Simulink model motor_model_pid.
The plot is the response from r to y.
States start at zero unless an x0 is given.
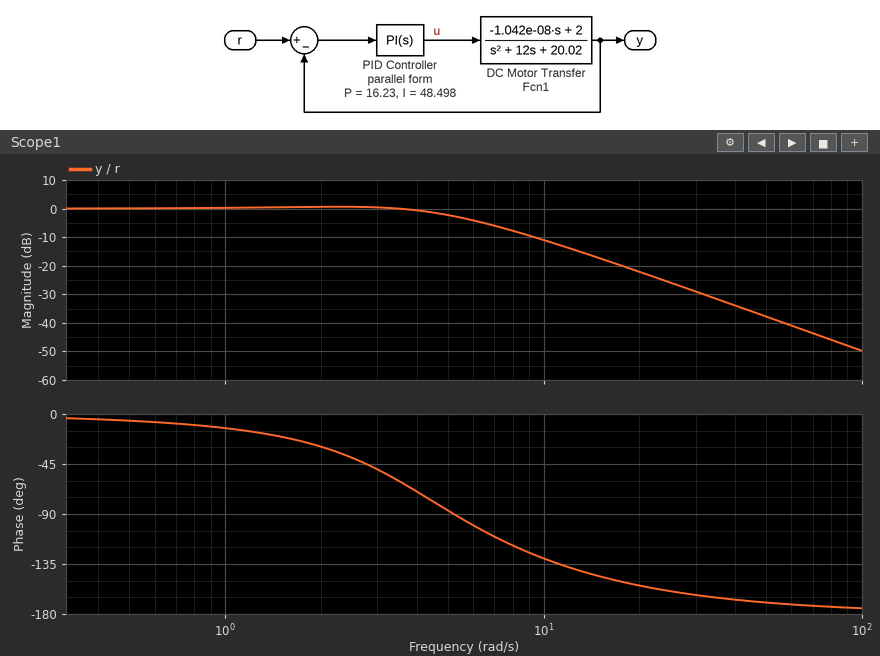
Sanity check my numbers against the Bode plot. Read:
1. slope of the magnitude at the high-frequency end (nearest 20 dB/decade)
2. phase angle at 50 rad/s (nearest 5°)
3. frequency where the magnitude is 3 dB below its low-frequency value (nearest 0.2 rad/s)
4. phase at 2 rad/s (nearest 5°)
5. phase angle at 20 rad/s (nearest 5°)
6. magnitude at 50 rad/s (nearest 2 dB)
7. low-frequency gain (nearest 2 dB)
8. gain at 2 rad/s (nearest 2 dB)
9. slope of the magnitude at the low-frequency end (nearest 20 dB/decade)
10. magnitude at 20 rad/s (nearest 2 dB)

-40 dB/decade
-170°
5.4 rad/s
-30°
-155°
-38 dB
0 dB
0 dB
0 dB/decade
-22 dB
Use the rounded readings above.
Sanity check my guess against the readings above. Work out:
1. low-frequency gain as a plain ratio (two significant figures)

1.0
